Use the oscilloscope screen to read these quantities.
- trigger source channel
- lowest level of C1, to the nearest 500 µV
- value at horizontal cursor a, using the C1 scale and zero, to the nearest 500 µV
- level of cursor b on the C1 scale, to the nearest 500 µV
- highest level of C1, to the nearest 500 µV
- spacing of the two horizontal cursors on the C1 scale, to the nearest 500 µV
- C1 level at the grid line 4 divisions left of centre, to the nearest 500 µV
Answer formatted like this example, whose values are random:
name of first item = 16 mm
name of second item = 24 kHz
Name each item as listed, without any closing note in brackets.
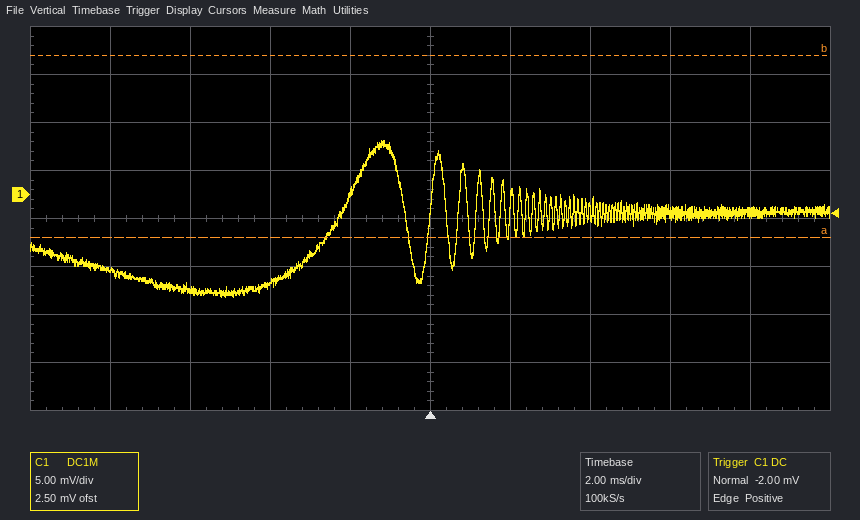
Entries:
trigger source channel = C1
lowest level of C1, to the nearest 500 µV = -10.5 mV
value at horizontal cursor a, using the C1 scale and zero, to the nearest 500 µV = -4.5 mV
level of cursor b on the C1 scale, to the nearest 500 µV = 14.5 mV
highest level of C1, to the nearest 500 µV = 5.5 mV
spacing of the two horizontal cursors on the C1 scale, to the nearest 500 µV = 19.0 mV
C1 level at the grid line 4 divisions left of centre, to the nearest 500 µV = -8.0 mV
